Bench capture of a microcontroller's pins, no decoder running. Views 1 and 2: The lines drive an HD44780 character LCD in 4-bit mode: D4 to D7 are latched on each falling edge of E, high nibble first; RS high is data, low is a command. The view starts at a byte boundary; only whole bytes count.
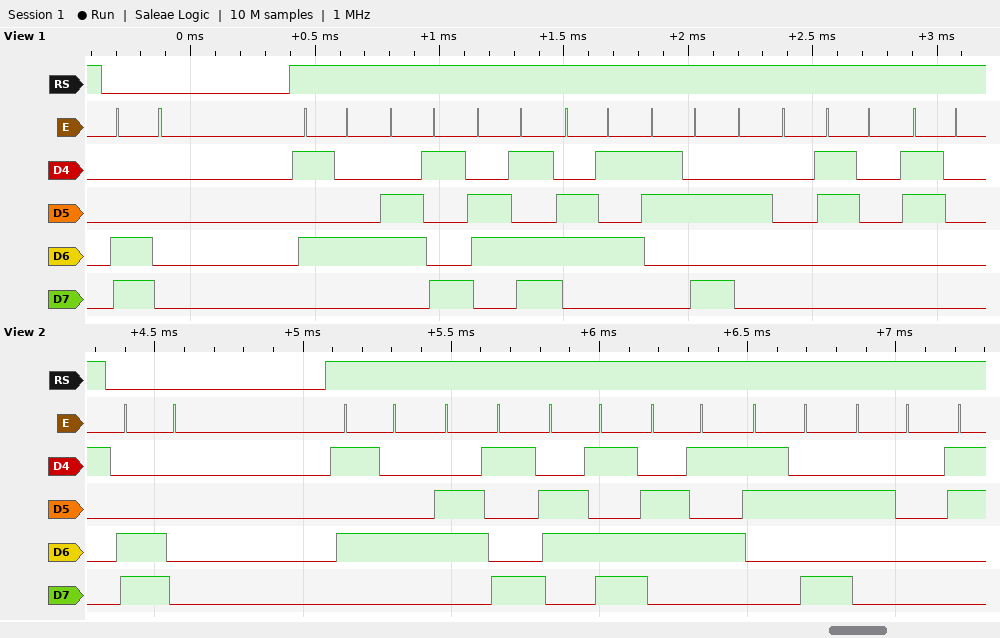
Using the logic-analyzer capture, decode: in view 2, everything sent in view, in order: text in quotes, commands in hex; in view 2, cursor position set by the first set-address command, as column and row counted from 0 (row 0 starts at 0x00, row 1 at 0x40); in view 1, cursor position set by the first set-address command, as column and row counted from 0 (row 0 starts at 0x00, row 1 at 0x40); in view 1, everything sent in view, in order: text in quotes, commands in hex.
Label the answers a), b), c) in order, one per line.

a) 0xC0 "Time: "
b) column 0, row 1
c) column 0, row 1
d) 0xC0 "Time: 00"
